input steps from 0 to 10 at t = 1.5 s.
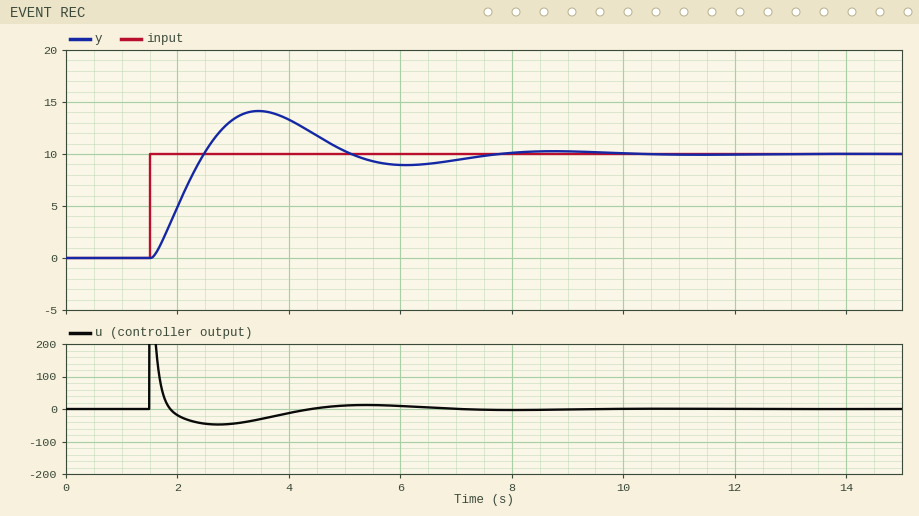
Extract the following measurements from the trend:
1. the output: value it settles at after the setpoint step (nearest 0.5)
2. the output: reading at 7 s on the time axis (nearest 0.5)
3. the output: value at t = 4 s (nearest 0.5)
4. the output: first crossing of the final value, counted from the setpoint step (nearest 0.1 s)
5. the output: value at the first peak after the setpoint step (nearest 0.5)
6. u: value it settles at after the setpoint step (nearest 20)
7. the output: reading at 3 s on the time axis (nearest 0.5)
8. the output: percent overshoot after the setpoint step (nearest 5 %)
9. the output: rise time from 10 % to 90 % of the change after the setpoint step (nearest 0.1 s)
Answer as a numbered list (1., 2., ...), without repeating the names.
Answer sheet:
1. 10.0
2. 9.5
3. 13.5
4. 1.0 s
5. 14.0
6. 0
7. 13.5
8. 40 %
9. 0.7 s
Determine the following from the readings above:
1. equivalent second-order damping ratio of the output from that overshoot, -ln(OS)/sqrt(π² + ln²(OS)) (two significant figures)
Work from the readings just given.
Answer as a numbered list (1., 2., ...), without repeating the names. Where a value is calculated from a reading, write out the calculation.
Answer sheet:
1. ln(0.4) = -0.916; 0.916 / sqrt(9.870 + 0.840) = 0.28
